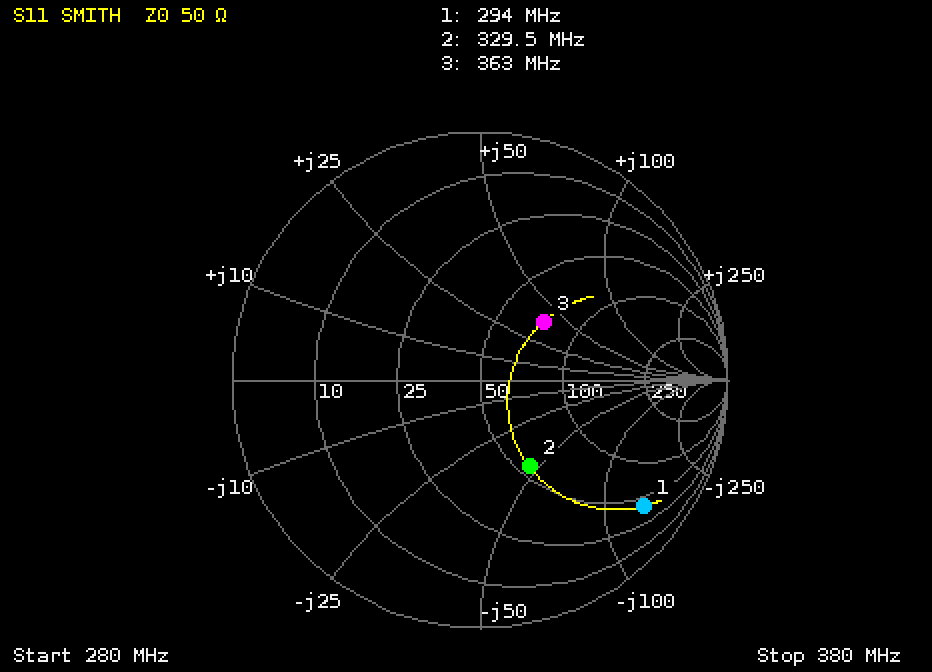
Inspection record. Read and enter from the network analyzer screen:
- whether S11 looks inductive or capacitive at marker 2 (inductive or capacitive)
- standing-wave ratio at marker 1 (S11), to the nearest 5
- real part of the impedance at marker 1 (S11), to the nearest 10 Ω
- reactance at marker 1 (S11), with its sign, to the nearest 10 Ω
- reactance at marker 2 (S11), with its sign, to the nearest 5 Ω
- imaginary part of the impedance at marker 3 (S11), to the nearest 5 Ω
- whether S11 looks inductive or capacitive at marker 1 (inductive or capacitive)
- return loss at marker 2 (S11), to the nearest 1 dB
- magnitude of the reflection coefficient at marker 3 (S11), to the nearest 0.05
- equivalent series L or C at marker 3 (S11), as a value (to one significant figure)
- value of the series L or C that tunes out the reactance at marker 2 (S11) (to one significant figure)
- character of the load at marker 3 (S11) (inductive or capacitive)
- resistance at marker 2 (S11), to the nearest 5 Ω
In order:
capacitive
10
40 Ω
-140 Ω
-45 Ω
+40 Ω
capacitive
8 dB
0.35
20 nH
20 nH
inductive
55 Ω
